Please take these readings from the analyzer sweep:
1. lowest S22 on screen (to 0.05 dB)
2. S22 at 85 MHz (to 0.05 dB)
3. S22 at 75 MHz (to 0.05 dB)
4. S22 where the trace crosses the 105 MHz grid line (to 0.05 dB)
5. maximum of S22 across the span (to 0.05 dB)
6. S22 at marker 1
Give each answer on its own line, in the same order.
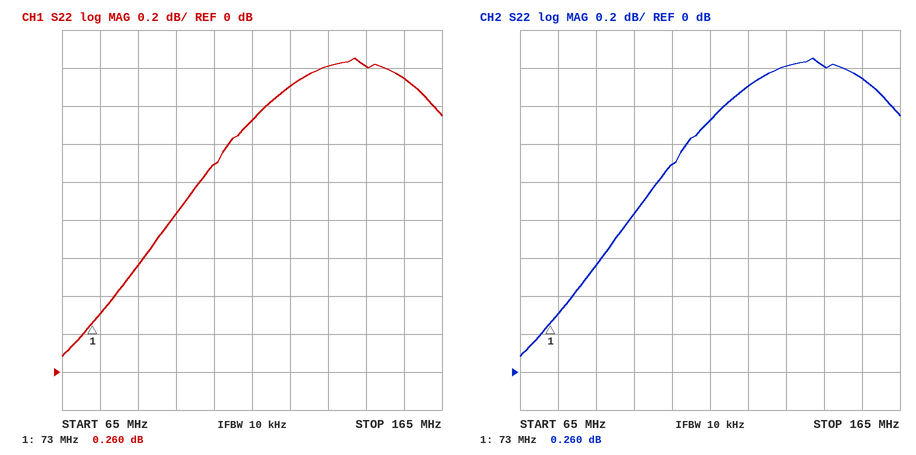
0.10 dB
0.55 dB
0.30 dB
1.10 dB
1.65 dB
0.260 dB
